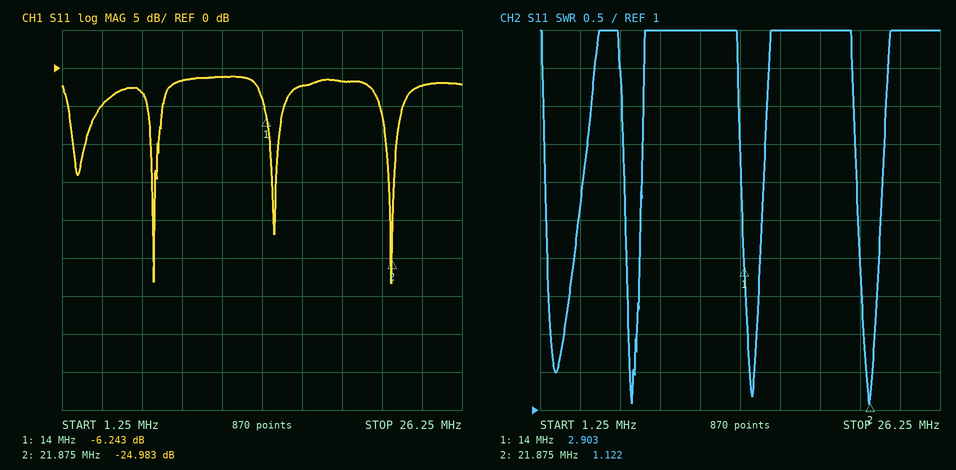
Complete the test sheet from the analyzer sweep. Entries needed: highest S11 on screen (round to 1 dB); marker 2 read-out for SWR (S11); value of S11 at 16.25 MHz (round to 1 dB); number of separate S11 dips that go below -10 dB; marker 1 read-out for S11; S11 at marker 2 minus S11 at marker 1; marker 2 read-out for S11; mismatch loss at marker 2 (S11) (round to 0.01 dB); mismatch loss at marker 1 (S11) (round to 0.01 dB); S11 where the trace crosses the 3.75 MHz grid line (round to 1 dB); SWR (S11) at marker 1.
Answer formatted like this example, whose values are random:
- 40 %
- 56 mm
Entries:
- -1 dB
- 1.122
- -2 dB
- 4
- -6.243 dB
- -18.740 dB
- -24.983 dB
- 0.01 dB
- 1.18 dB
- -5 dB
- 2.903
